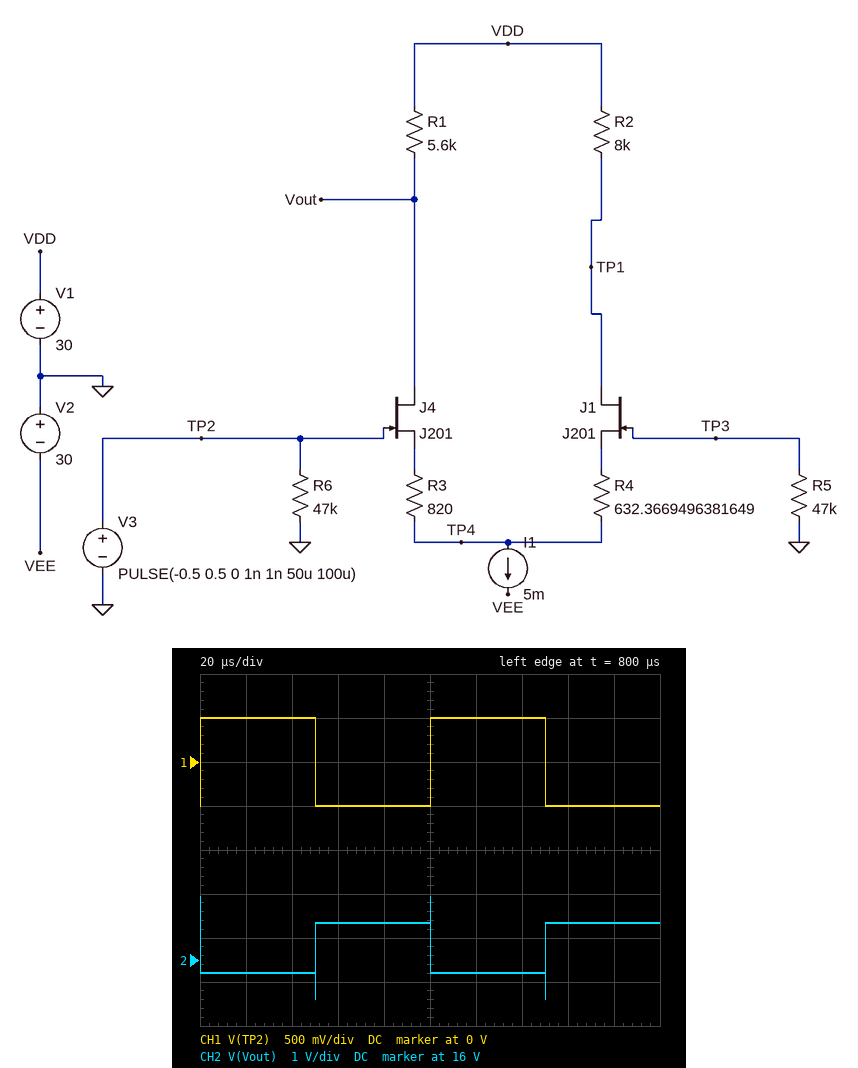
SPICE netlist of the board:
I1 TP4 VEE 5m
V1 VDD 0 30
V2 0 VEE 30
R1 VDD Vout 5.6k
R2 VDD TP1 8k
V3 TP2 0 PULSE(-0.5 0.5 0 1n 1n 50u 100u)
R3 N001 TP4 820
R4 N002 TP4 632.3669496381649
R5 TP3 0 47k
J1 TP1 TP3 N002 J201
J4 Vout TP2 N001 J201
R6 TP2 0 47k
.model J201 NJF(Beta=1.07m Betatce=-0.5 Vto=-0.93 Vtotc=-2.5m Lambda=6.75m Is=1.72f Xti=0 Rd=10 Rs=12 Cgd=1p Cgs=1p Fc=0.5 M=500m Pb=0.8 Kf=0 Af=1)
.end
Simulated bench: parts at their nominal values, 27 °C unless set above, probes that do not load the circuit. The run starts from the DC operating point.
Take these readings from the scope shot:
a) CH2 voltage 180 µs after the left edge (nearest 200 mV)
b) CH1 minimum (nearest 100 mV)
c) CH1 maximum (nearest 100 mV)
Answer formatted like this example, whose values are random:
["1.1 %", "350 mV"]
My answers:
["16.8 V", "-500 mV", "500 mV"]
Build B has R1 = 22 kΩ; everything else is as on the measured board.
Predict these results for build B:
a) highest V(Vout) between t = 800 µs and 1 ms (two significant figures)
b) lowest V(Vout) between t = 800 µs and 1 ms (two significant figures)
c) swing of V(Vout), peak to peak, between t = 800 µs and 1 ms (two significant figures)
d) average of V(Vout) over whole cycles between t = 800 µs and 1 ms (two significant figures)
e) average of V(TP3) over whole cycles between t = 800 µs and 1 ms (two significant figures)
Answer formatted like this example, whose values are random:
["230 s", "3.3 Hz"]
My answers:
["270 mV", "-730 mV", "1.0 V", "-230 mV", "-470 mV"]
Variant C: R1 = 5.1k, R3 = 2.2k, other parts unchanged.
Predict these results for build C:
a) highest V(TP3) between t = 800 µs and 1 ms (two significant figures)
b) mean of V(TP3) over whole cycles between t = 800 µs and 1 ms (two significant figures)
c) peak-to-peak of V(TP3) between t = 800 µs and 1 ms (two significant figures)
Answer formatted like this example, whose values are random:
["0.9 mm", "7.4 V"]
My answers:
["-2.3 V", "-2.7 V", "820 mV"]
